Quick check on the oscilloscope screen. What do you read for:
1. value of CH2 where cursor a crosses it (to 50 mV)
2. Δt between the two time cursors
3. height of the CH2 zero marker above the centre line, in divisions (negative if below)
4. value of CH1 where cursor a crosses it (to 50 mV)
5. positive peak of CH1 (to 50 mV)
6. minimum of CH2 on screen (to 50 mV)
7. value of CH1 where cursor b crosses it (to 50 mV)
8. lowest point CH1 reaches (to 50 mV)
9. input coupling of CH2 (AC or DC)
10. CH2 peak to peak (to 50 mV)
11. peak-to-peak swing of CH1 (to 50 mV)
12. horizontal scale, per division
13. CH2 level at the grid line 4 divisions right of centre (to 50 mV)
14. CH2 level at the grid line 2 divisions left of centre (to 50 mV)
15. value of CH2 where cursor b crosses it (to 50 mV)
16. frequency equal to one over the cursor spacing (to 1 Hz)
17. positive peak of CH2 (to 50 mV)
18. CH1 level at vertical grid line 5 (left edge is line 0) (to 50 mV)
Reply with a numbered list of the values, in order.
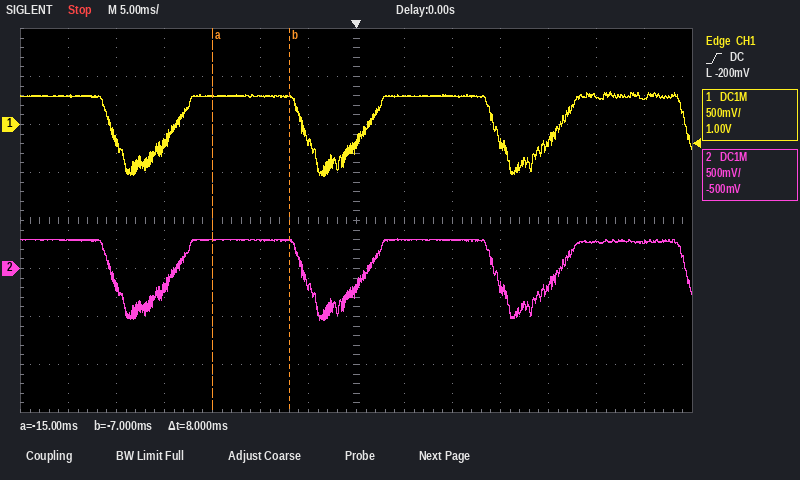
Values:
1. 300 mV
2. 8 ms
3. -1.0 div
4. 300 mV
5. 350 mV
6. -550 mV
7. 300 mV
8. -550 mV
9. DC
10. 850 mV
11. 900 mV
12. 5 ms
13. -200 mV
14. 300 mV
15. 300 mV
16. 125 Hz
17. 300 mV
18. 300 mV
